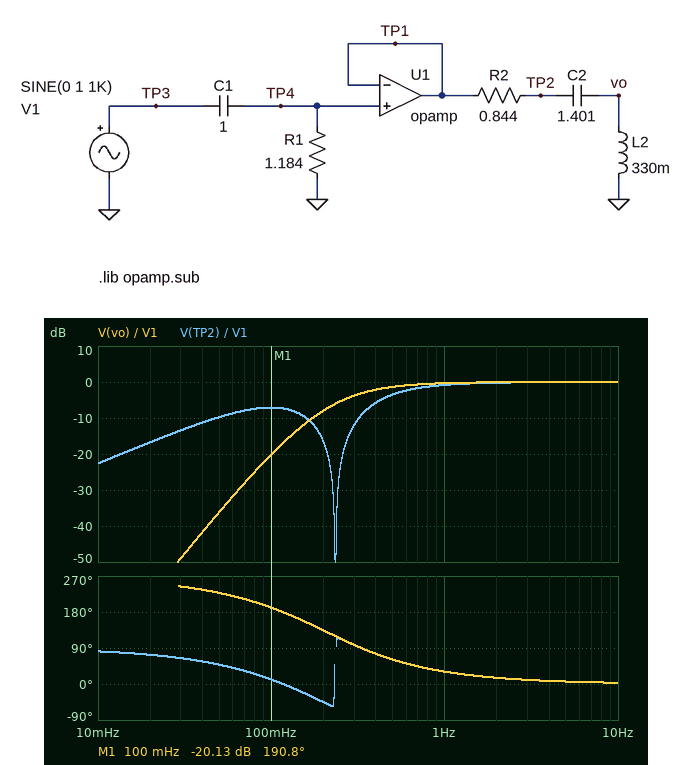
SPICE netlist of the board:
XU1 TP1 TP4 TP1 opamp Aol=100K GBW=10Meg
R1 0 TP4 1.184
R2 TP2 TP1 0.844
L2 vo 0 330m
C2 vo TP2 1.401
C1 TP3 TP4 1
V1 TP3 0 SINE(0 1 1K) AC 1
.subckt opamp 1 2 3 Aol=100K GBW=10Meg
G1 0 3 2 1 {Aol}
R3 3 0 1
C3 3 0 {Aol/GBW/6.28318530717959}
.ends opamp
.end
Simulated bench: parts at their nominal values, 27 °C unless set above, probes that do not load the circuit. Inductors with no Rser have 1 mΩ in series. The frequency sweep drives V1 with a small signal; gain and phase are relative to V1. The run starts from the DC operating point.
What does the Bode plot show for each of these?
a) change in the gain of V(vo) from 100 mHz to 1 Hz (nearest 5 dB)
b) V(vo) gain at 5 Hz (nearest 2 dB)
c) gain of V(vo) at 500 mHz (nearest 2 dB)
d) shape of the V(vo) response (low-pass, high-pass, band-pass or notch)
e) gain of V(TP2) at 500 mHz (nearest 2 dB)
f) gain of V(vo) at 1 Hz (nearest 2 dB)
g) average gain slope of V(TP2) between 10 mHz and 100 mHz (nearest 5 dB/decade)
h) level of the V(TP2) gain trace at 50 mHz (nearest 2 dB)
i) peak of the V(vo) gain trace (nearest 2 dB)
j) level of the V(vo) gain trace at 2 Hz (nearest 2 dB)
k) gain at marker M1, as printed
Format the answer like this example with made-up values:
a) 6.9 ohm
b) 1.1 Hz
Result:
a) 20 dB
b) 0 dB
c) -2 dB
d) high-pass
e) -4 dB
f) 0 dB
g) 15 dB/decade
h) -10 dB
i) 0 dB
j) 0 dB
k) -20.13 dB
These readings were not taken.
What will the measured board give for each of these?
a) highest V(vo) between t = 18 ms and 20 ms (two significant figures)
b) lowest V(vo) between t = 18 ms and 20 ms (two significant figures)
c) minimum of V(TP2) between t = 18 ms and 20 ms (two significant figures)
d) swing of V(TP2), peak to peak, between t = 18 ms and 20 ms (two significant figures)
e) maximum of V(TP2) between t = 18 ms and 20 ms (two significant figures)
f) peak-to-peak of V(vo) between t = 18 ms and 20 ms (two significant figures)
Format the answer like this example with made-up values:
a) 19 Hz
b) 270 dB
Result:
a) 1.0 V
b) -1.0 V
c) -1.0 V
d) 2.0 V
e) 1.0 V
f) 2.0 V
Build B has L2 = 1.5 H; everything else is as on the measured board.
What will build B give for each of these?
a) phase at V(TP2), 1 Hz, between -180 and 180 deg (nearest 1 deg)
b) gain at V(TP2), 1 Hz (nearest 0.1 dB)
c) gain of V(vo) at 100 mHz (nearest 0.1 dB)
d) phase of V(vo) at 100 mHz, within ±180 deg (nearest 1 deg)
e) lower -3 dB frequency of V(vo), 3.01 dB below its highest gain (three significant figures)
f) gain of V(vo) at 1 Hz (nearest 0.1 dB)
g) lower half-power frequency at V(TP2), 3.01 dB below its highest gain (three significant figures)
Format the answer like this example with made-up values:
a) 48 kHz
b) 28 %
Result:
a) 13 deg
b) -0.1 dB
c) -3.8 dB
d) 156 deg
e) 104 mHz
f) 0 dB
g) 203 mHz
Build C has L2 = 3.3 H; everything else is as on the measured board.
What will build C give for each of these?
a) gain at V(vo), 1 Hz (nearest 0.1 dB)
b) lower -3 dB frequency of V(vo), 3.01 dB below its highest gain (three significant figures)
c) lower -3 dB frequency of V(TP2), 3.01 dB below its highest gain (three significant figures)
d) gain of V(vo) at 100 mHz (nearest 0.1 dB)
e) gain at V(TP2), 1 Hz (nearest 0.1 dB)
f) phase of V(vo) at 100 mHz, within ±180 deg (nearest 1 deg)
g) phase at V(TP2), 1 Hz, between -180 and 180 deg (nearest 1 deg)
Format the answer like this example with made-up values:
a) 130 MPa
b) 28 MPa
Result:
a) 0 dB
b) 67.6 mHz
c) 152 mHz
d) -0.2 dB
e) -0.1 dB
f) 95 deg
g) 10 deg
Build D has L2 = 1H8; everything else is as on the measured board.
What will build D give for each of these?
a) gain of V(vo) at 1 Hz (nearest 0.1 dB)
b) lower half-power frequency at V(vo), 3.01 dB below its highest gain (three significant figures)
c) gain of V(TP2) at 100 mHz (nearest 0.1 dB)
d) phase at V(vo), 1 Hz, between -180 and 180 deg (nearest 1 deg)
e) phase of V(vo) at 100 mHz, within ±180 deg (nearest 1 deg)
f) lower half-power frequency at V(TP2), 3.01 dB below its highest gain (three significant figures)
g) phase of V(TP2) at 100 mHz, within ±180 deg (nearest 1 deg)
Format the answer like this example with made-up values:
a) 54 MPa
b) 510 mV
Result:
a) 0 dB
b) 93.8 mHz
c) -48.8 dB
d) 12 deg
e) 144 deg
f) 187 mHz
g) -25 deg
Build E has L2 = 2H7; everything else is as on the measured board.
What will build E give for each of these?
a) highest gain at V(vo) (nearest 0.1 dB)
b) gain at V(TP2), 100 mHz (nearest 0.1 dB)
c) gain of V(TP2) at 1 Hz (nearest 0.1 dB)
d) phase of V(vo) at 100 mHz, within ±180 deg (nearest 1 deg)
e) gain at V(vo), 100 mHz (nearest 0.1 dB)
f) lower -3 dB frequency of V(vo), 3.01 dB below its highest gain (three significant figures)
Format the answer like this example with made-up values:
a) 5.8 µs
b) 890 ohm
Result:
a) 0 dB
b) -9.6 dB
c) -0.1 dB
d) 110 deg
e) 0 dB
f) 75.1 mHz
